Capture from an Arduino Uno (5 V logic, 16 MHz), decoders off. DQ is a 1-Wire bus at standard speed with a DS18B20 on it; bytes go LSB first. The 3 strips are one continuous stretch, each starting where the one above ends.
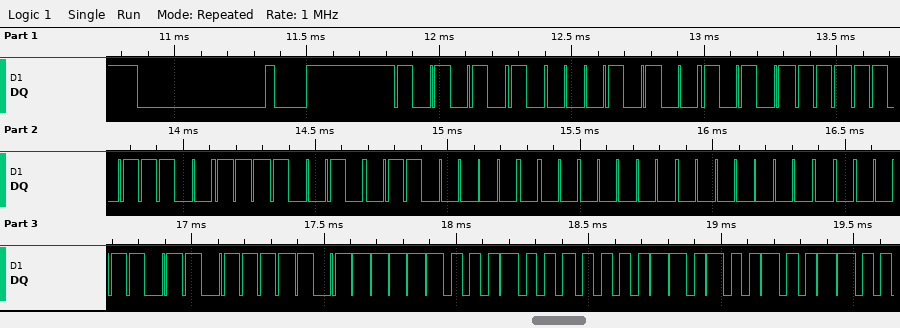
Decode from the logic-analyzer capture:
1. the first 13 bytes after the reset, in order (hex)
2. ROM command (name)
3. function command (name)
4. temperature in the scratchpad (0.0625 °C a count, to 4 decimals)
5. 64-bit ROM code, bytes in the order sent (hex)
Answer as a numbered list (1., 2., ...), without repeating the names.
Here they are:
1. 55 28 F5 3B 4F 06 00 00 D8 BE 1F 01 4B
2. Match ROM
3. Read Scratchpad
4. 17.9375 °C
5. 28 F5 3B 4F 06 00 00 D8
